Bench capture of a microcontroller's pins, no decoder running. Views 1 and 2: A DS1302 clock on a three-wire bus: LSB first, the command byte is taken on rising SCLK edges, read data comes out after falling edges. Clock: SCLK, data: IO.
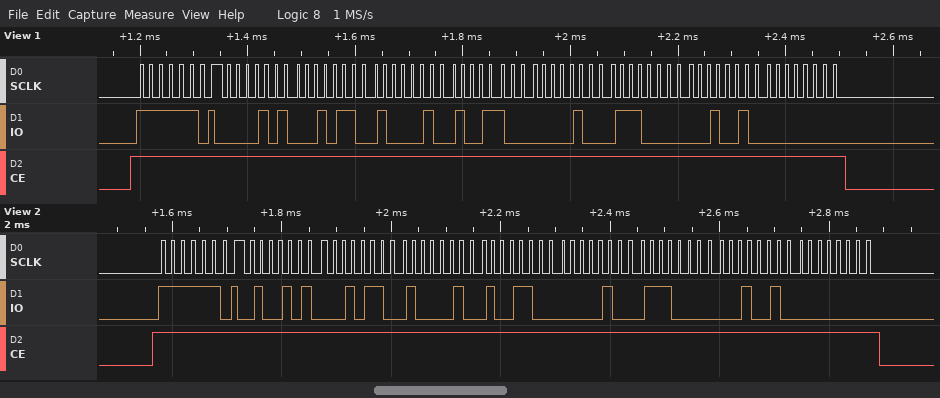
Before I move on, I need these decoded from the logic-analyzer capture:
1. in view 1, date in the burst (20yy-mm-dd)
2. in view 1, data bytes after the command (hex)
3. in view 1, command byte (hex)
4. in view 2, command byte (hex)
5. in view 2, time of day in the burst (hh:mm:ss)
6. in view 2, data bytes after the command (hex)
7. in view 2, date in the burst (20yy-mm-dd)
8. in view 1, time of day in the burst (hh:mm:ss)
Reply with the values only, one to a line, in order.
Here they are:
2024-10-19
50 34 21 19 10 07 24 00
0xBF
0xBF
21:34:52
52 34 21 19 10 07 24 00
2024-10-19
21:34:50
